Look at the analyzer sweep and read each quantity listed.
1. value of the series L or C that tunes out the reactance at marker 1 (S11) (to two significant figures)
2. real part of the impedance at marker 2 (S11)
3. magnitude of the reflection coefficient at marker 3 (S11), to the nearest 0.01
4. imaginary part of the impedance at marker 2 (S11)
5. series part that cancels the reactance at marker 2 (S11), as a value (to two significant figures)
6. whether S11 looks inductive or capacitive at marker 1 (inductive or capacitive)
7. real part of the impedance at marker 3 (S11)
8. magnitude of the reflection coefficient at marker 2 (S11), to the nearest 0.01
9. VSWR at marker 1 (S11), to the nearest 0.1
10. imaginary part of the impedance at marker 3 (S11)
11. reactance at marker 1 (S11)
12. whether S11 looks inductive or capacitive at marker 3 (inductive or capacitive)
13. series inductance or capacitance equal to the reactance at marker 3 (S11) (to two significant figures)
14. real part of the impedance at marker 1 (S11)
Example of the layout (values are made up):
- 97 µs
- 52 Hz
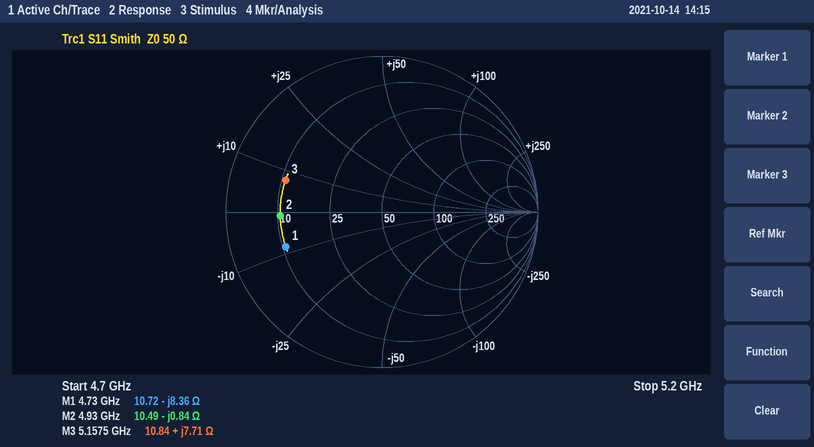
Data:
- 280 pH
- 10.49 Ω
- 0.65
- -0.84 Ω
- 27 pH
- capacitive
- 10.84 Ω
- 0.65
- 4.8
- +7.71 Ω
- -8.36 Ω
- inductive
- 240 pH
- 10.72 Ω
